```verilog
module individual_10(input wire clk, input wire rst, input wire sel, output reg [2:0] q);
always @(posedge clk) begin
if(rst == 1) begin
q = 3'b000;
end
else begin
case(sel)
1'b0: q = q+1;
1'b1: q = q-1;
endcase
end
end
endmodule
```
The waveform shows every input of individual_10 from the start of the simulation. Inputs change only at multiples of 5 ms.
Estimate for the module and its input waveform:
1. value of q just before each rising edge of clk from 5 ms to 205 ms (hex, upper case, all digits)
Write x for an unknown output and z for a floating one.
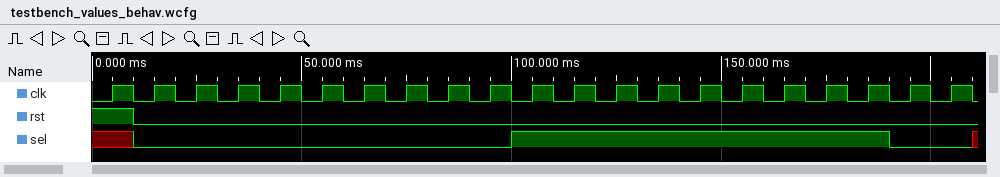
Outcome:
x, 0, 1, 2, 3, 4, 5, 6, 7, 0, 1, 0, 7, 6, 5, 4, 3, 2, 1, 0, 1
